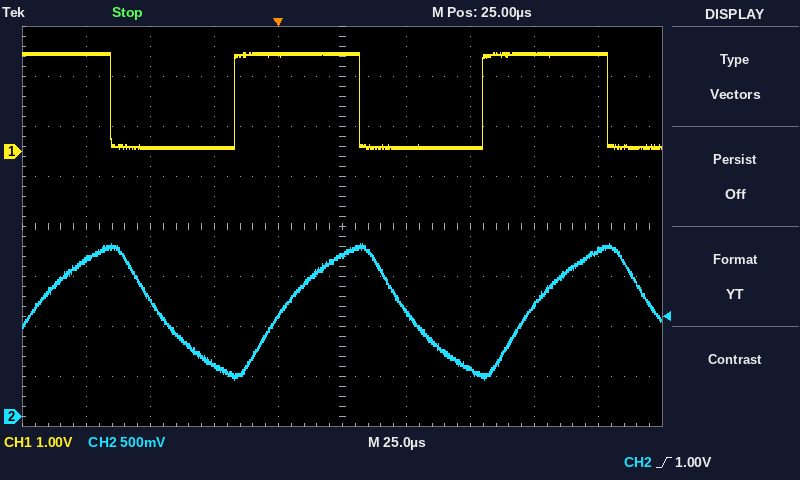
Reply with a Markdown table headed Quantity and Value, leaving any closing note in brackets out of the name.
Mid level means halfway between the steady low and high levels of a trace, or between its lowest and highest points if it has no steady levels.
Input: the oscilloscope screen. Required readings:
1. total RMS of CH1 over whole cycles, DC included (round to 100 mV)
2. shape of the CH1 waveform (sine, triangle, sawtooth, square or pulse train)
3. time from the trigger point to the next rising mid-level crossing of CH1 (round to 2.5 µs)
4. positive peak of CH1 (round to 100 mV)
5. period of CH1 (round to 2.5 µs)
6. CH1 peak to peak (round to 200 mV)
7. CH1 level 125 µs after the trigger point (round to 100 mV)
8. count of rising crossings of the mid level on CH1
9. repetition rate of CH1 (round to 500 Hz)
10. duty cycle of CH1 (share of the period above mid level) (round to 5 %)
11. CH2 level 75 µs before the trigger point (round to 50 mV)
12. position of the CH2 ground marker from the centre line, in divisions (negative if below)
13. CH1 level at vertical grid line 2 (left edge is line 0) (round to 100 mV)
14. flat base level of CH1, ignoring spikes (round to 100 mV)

| Quantity | Value |
|---|---|
| total RMS of CH1 over whole cycles, DC included | 1.4 V |
| shape of the CH1 waveform | square |
| time from the trigger point to the next rising mid-level crossing of CH1 | 80.0 µs |
| positive peak of CH1 | 2.0 V |
| period of CH1 | 97.5 µs |
| CH1 peak to peak | 2.0 V |
| CH1 level 125 µs after the trigger point | 2.0 V |
| count of rising crossings of the mid level on CH1 | 2 |
| repetition rate of CH1 | 10.5 kHz |
| duty cycle of CH1 (share of the period above mid level) | 50 % |
| CH2 level 75 µs before the trigger point | 1.55 V |
| position of the CH2 ground marker from the centre line, in divisions | -3.8 div |
| CH1 level at vertical grid line 2 (left edge is line 0) | 100 mV |
| flat base level of CH1, ignoring spikes | 100 mV |
